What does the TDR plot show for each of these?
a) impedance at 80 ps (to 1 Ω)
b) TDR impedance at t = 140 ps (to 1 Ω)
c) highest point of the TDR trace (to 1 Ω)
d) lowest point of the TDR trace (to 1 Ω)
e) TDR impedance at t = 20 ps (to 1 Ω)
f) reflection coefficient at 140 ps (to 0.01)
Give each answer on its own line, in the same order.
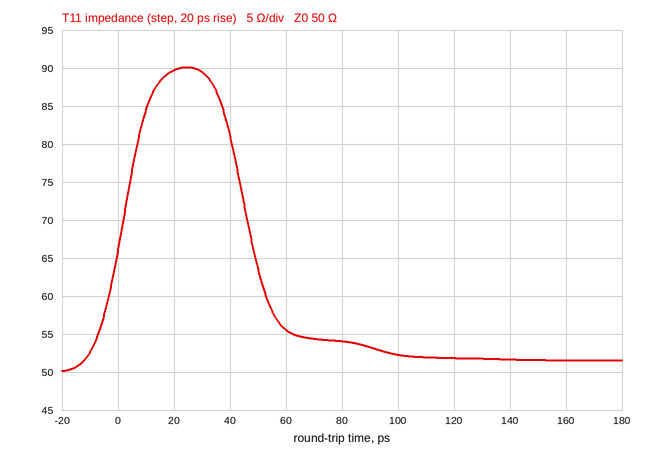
54 Ω
52 Ω
90 Ω
50 Ω
90 Ω
+0.02
